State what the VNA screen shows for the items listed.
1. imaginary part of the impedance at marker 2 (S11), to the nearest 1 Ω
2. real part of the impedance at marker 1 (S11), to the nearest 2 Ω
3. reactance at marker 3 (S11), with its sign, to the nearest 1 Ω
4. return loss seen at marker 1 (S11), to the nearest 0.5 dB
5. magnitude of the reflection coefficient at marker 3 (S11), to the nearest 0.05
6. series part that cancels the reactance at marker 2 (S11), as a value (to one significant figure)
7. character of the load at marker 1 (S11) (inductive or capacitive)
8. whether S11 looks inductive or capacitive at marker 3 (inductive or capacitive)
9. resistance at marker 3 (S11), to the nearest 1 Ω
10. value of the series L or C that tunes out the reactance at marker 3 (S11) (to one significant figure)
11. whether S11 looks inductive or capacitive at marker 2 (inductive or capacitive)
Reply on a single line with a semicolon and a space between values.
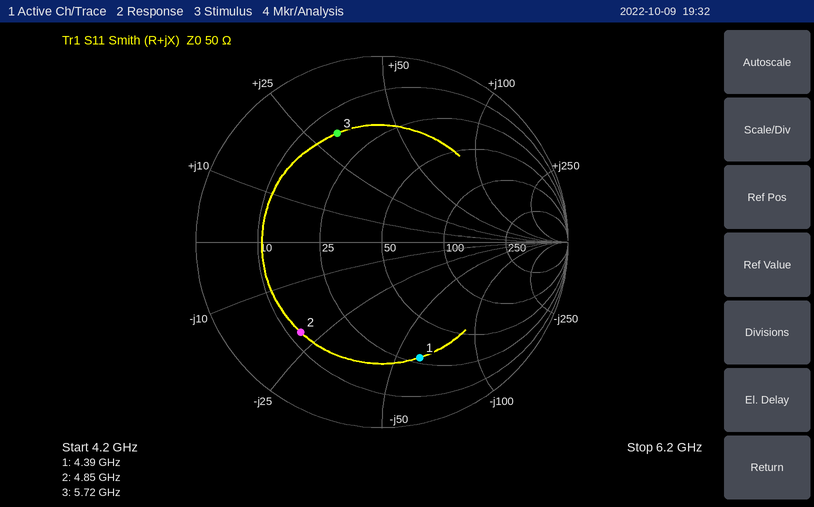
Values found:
-21 Ω; 28 Ω; +31 Ω; 3.5 dB; 0.65; 700 pH; capacitive; inductive; 16 Ω; 900 fF; capacitive
